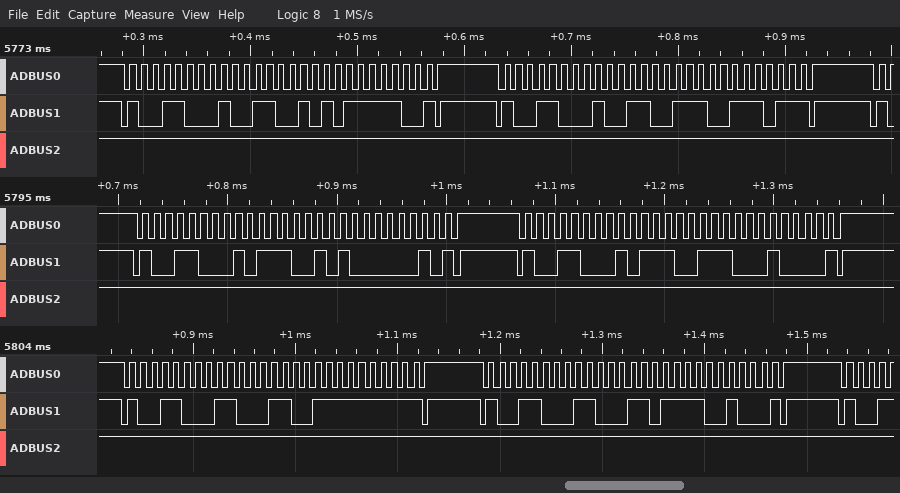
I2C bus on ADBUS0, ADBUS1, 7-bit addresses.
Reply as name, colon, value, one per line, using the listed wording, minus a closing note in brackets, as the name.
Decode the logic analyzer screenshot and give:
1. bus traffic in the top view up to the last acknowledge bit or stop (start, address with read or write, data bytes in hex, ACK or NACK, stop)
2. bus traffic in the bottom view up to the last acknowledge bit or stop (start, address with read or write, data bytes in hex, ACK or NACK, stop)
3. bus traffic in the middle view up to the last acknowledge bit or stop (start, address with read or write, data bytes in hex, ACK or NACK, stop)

bus traffic in the top view up to the last acknowledge bit or stop: start, address 4C write NACK, 32 NACK, 7C NACK, stop, start, address 4C write NACK, 33 NACK, 3B NACK, stop
bus traffic in the bottom view up to the last acknowledge bit or stop: start, address 4C write NACK, 8C NACK, FF NACK, stop, start, address 4C write NACK, 8D NACK, C8 NACK, stop
bus traffic in the middle view up to the last acknowledge bit or stop: start, address 4C write NACK, 72 NACK, 02 NACK, stop, start, address 4C write NACK, 73 NACK, 10 NACK, stop
